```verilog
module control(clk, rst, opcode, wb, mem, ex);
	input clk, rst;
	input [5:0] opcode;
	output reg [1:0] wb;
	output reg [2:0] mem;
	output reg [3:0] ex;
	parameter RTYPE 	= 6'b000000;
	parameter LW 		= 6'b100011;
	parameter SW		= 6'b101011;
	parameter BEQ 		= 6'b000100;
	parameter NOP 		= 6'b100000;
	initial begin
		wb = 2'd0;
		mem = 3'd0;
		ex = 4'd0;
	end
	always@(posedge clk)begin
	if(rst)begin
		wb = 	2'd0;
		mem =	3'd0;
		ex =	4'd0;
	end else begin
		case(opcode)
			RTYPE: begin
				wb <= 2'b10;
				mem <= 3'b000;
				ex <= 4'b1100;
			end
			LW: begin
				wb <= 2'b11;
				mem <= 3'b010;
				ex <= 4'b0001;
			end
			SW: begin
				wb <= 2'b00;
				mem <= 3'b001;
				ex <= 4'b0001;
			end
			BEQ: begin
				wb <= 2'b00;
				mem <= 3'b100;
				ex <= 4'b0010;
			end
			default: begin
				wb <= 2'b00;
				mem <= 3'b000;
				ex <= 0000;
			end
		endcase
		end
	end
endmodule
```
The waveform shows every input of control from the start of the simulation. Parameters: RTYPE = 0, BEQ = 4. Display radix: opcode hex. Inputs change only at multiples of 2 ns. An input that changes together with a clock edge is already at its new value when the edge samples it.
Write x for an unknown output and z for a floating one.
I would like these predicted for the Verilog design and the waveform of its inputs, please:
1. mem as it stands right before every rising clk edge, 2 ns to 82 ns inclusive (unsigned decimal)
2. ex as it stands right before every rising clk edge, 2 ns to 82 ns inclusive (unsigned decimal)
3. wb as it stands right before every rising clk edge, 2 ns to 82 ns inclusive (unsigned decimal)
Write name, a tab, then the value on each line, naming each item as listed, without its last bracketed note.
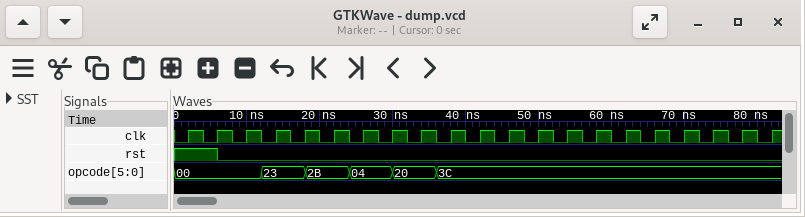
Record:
mem as it stands right before every rising clk edge, 2 ns to 82 ns inclusive	0, 0, 0, 0, 2, 1, 1, 4, 0, 0, 0, 0, 0, 0, 0, 0, 0, 0, 0, 0, 0
ex as it stands right before every rising clk edge, 2 ns to 82 ns inclusive	0, 0, 12, 12, 1, 1, 1, 2, 0, 0, 0, 0, 0, 0, 0, 0, 0, 0, 0, 0, 0
wb as it stands right before every rising clk edge, 2 ns to 82 ns inclusive	0, 0, 2, 2, 3, 0, 0, 0, 0, 0, 0, 0, 0, 0, 0, 0, 0, 0, 0, 0, 0
